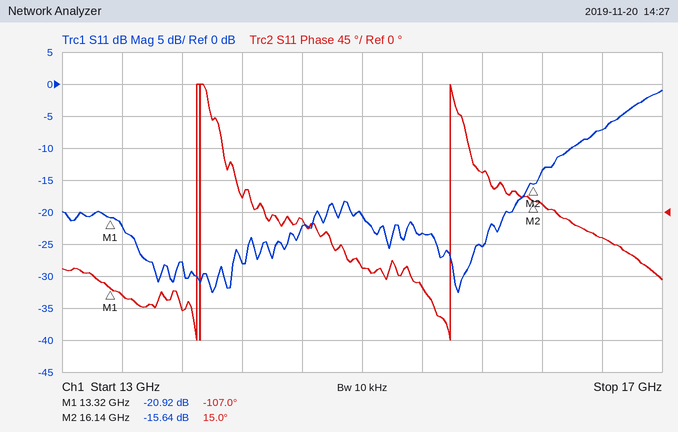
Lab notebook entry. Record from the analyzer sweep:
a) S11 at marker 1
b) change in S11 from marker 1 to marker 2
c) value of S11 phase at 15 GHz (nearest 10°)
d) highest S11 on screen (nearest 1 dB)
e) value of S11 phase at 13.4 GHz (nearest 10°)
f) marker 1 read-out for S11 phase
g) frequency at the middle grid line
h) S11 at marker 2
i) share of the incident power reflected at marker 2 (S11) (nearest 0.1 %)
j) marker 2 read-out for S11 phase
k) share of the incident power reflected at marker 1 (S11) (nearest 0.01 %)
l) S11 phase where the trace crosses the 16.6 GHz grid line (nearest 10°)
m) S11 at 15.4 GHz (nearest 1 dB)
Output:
-20.92 dB
5.28 dB
-80°
-1 dB
-120°
-107.0°
15 GHz
-15.64 dB
2.7 %
15.0°
0.81 %
-40°
-23 dB
